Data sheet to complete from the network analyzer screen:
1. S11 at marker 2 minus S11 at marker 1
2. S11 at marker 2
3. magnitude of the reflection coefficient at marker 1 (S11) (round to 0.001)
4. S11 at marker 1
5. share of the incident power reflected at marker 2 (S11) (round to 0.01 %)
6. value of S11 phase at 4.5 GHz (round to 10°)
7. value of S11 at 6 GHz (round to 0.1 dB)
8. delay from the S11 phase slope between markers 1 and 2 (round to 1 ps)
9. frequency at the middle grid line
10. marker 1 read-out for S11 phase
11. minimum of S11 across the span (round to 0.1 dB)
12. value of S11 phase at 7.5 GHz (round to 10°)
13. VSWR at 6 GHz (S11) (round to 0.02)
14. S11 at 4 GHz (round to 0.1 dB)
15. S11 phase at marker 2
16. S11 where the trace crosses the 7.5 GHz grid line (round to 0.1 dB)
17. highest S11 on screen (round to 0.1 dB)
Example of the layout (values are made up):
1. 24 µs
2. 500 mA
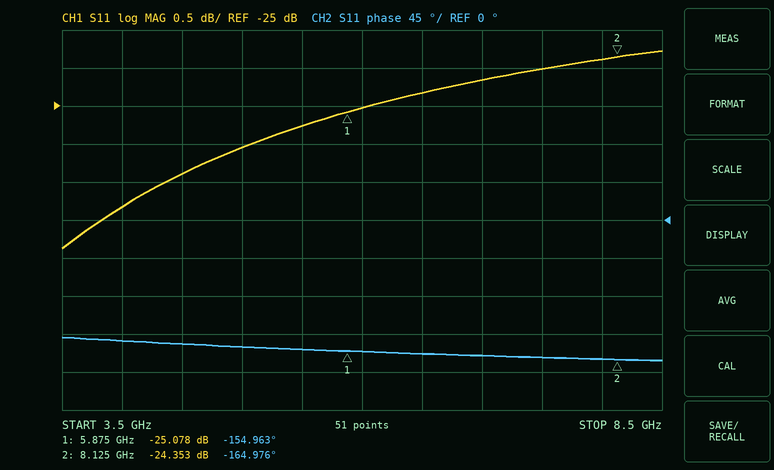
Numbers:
1. 0.725 dB
2. -24.353 dB
3. 0.056
4. -25.078 dB
5. 0.37 %
6. -150°
7. -25.0 dB
8. 12 ps
9. 6 GHz
10. -154.963°
11. -26.9 dB
12. -160°
13. 1.12
14. -26.3 dB
15. -164.976°
16. -24.5 dB
17. -24.3 dB
